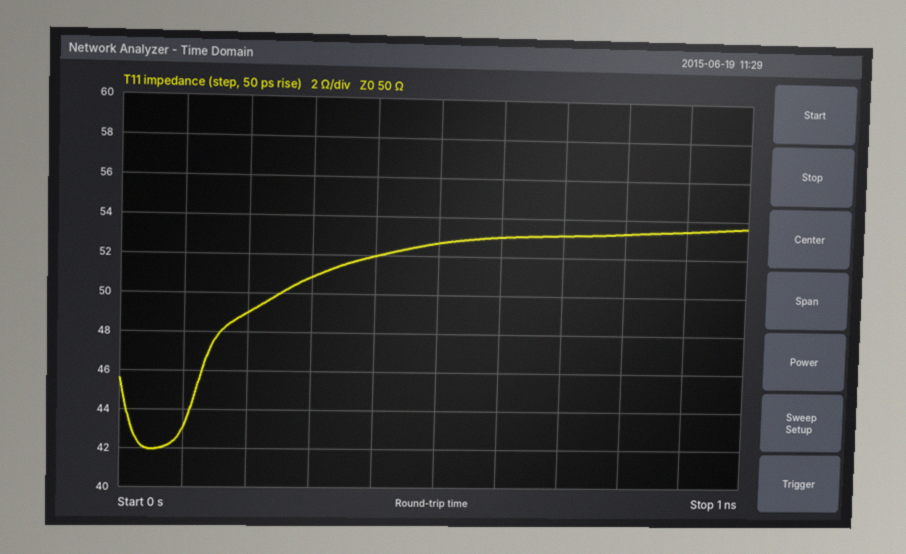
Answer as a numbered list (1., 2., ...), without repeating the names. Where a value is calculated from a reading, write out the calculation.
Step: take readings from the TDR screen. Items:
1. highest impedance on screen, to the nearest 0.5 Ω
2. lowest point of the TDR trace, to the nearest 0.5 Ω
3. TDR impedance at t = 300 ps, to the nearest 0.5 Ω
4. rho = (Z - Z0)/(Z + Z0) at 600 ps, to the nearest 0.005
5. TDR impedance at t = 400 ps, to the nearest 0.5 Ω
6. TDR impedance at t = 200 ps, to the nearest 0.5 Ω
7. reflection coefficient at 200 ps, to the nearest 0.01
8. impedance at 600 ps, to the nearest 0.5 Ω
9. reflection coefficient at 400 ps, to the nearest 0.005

1. 53.5 Ω
2. 42.0 Ω
3. 51.0 Ω
4. (53 − 50)/(53 + 50) ≈ +0.0291, so +0.030 to the nearest 0.005
5. 52.0 Ω
6. 49.0 Ω
7. (49 − 50)/(49 + 50) ≈ -0.01
8. 53.0 Ω
9. (52 − 50)/(52 + 50) ≈ +0.020
